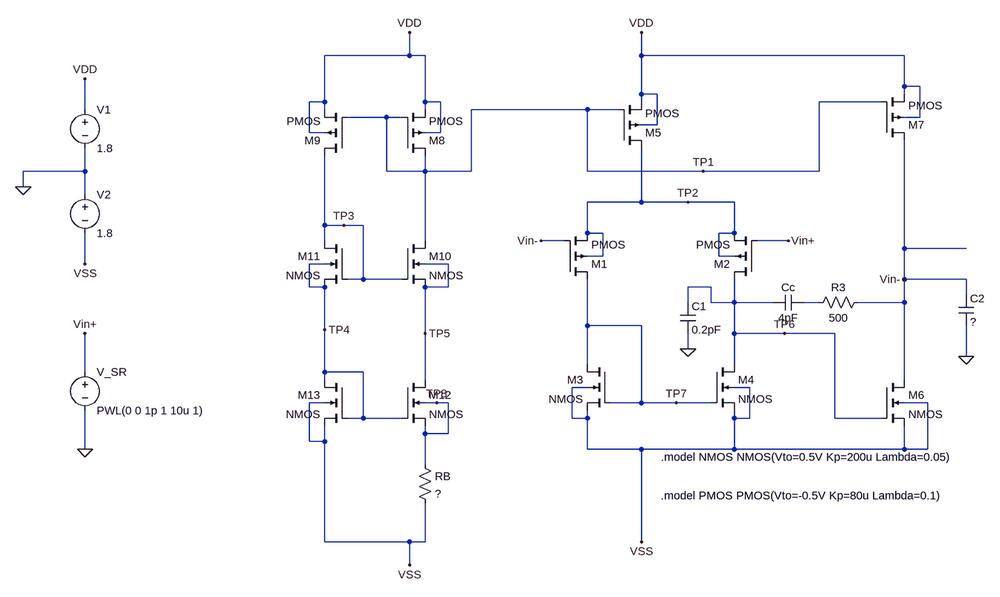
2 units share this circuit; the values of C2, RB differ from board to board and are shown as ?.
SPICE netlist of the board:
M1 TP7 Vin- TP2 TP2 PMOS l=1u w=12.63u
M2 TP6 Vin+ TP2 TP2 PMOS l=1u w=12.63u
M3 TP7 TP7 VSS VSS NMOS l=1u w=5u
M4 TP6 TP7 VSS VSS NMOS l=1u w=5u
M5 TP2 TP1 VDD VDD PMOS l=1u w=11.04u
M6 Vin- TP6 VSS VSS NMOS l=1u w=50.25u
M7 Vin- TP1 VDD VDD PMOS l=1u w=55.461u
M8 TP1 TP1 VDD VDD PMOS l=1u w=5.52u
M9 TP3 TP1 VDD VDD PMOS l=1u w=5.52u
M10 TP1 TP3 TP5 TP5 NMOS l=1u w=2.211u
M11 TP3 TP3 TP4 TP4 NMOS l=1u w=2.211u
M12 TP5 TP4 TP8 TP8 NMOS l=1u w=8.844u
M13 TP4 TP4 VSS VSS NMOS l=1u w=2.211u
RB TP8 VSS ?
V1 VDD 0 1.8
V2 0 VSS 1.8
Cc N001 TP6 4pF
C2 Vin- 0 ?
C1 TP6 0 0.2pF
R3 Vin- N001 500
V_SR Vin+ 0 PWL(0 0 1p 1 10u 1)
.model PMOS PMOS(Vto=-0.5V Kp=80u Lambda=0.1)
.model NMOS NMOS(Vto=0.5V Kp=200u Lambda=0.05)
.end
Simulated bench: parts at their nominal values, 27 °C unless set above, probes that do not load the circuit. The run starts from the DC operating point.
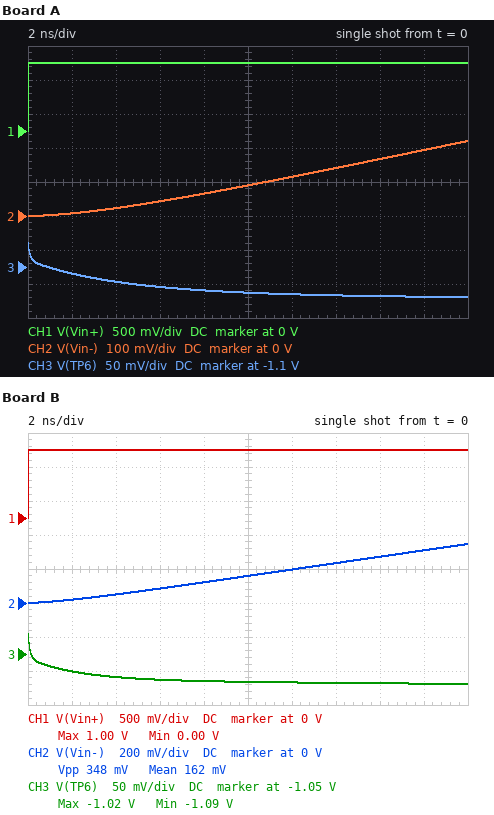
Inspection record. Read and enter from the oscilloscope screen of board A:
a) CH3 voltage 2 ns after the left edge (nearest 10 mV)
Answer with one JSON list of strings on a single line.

["-1.11 V"]
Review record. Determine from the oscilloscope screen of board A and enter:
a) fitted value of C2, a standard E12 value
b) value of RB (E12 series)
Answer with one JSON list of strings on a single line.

["8.2 pF", "6.8 kΩ"]
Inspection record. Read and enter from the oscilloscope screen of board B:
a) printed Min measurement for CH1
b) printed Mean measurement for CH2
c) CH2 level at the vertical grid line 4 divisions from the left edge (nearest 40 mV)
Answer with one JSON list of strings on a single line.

["0.00 V", "162 mV", "120 mV"]
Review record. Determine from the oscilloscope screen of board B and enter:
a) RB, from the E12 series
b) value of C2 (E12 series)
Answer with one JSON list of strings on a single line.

["5.6 kΩ", "5.6 pF"]
